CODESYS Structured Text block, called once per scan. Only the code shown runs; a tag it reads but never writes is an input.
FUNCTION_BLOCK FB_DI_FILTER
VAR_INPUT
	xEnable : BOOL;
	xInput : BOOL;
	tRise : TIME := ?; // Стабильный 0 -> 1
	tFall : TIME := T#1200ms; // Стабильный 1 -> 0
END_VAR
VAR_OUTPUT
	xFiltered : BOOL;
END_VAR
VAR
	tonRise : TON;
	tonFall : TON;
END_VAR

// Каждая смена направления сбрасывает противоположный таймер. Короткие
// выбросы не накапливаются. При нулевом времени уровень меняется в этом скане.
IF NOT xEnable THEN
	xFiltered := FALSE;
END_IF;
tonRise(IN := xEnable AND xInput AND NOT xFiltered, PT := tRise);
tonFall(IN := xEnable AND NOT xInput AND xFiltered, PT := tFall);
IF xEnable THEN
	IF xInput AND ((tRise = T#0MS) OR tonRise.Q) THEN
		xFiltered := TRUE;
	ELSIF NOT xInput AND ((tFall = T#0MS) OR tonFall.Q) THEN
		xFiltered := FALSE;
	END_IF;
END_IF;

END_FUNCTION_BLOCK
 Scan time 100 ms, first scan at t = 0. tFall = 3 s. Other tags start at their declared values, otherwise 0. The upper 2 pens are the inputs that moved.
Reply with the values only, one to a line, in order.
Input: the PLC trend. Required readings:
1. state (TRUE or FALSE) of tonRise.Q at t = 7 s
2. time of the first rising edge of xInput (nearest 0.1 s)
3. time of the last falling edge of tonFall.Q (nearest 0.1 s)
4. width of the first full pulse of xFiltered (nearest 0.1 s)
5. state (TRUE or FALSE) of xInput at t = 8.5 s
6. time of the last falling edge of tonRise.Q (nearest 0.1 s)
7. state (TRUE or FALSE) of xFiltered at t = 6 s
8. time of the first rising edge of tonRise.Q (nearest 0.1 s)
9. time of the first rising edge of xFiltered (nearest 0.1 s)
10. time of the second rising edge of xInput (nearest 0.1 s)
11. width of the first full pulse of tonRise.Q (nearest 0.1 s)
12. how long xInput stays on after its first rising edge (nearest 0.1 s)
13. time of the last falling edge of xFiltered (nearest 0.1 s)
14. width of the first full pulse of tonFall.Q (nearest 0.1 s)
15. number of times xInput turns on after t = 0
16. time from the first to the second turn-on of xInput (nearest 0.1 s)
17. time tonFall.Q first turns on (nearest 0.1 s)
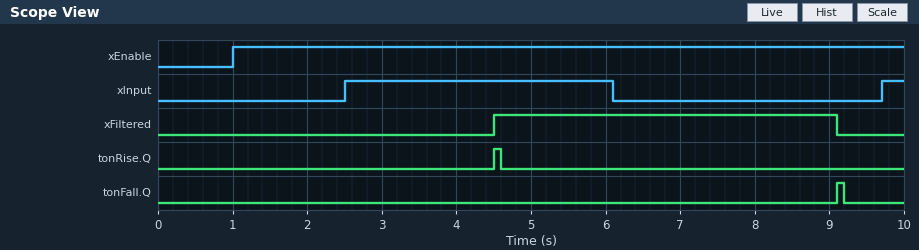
FALSE
2.5 s
9.2 s
4.6 s
FALSE
4.6 s
TRUE
4.5 s
4.5 s
9.7 s
0.1 s
3.6 s
9.1 s
0.1 s
2
7.2 s
9.1 s
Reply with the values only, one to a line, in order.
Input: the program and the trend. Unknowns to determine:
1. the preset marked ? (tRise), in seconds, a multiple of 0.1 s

2.0 s
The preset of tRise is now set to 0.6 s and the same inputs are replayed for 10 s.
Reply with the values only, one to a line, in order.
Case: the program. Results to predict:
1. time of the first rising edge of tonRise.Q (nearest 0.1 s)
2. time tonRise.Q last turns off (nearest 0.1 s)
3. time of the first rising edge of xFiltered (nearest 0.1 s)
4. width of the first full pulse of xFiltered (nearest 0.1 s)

3.1 s
3.2 s
3.1 s
6.0 s
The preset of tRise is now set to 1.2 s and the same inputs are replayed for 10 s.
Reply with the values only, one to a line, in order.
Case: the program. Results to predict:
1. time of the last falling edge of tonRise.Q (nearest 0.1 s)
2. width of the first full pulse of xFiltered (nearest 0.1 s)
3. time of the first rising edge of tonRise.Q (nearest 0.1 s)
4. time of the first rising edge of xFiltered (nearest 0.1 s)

3.8 s
5.4 s
3.7 s
3.7 s
